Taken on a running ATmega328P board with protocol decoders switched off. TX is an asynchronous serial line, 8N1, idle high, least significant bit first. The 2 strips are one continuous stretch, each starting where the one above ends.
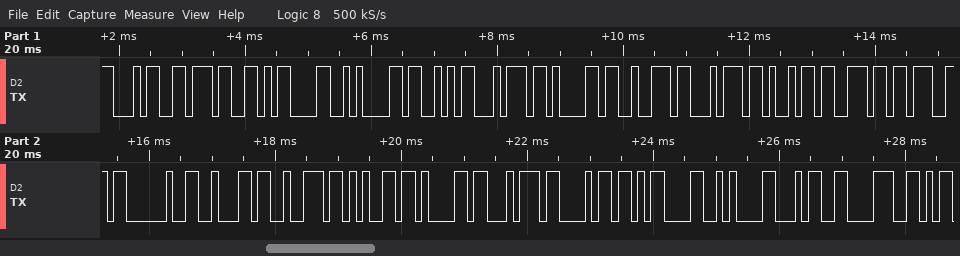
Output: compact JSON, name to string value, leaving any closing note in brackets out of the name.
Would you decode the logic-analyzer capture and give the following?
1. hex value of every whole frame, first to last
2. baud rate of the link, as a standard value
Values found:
{"hex value of every whole frame, first to last": "34 37 0D 0A 53 74 61 72 74 69 6E 67 20 62 72 65 61 74 68 0D 0A 34 38", "baud rate of the link, as a standard value": "9600 baud"}
